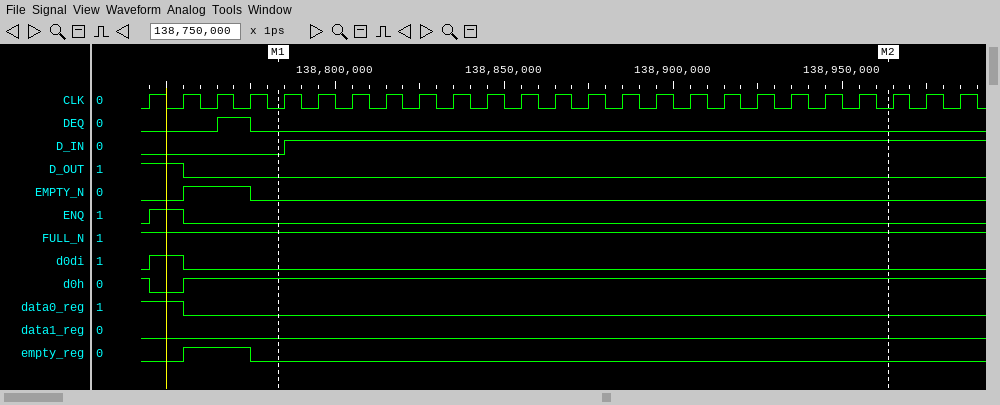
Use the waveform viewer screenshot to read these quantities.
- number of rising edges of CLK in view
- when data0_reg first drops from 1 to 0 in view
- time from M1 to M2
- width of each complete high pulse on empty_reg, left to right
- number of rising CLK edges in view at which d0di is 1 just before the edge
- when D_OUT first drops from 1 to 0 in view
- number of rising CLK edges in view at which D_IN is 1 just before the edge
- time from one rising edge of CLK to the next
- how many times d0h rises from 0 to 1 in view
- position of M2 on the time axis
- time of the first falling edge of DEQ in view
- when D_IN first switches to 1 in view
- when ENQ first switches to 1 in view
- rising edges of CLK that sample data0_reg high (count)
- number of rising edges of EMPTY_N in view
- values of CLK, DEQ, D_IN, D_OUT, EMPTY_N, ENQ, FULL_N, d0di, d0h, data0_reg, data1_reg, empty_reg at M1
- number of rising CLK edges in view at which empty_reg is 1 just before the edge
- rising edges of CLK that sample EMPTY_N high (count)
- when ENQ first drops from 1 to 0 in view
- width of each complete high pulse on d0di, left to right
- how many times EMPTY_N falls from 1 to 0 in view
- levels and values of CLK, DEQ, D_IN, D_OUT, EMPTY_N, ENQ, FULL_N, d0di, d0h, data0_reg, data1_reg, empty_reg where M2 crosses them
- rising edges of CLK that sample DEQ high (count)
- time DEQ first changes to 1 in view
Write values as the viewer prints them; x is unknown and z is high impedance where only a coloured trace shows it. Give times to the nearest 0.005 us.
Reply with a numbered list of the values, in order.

1. 25
2. 138.755 us
3. 0.18 us
4. 0.02 us
5. 1
6. 138.755 us
7. 20
8. 0.01 us
9. 1
10. 138.965 us
11. 138.775 us
12. 138.785 us
13. 138.745 us
14. 2
15. 1
16. CLK=0, DEQ=0, D_IN=0, D_OUT=0, EMPTY_N=0, ENQ=0, FULL_N=1, d0di=0, d0h=1, data0_reg=0, data1_reg=0, empty_reg=0
17. 2
18. 2
19. 138.755 us
20. 0.01 us
21. 1
22. CLK=0, DEQ=0, D_IN=1, D_OUT=0, EMPTY_N=0, ENQ=0, FULL_N=1, d0di=0, d0h=1, data0_reg=0, data1_reg=0, empty_reg=0
23. 1
24. 138.765 us
